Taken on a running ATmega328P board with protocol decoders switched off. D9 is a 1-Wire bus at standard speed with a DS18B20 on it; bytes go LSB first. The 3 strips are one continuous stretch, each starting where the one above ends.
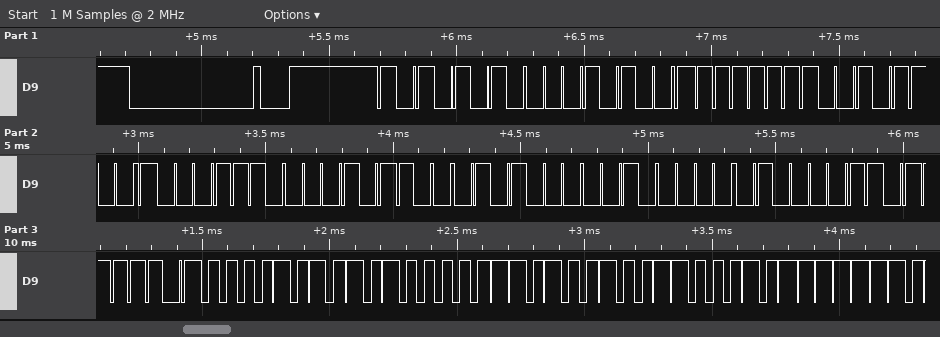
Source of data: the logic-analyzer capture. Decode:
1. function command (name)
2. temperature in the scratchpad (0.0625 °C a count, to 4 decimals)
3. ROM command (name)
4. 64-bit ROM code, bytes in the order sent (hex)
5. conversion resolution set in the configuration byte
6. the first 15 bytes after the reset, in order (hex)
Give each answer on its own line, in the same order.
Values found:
Read Scratchpad
85.0000 °C
Match ROM
28 FF 34 71 68 14 04 C2
12 bits
55 28 FF 34 71 68 14 04 C2 BE 50 05 4B 46 7F
